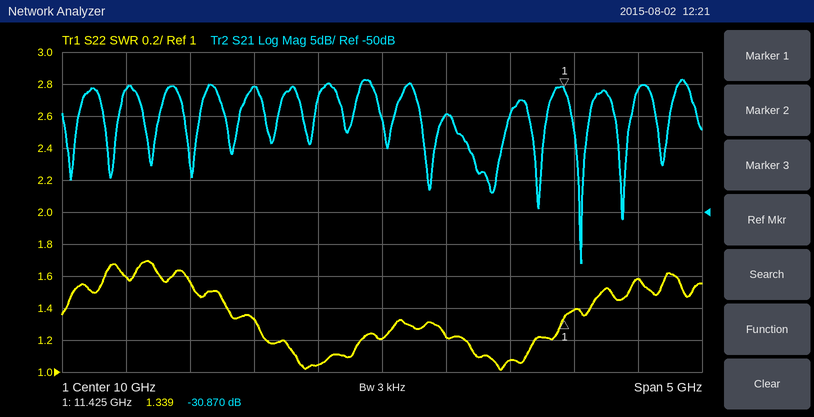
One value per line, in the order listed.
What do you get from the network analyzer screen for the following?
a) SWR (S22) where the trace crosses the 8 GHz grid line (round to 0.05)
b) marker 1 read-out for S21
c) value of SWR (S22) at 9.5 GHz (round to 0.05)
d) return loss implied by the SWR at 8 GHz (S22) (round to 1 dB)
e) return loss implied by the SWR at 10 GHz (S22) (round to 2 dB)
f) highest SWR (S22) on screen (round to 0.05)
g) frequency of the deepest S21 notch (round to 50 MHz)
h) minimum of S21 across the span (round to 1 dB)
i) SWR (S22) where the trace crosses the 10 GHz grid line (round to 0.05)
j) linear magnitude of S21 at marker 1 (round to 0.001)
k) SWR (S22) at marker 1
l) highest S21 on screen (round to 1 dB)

1.60
-30.870 dB
1.05
13 dB
20 dB
1.70
11.55 GHz
-58 dB
1.20
0.029
1.339
-29 dB
